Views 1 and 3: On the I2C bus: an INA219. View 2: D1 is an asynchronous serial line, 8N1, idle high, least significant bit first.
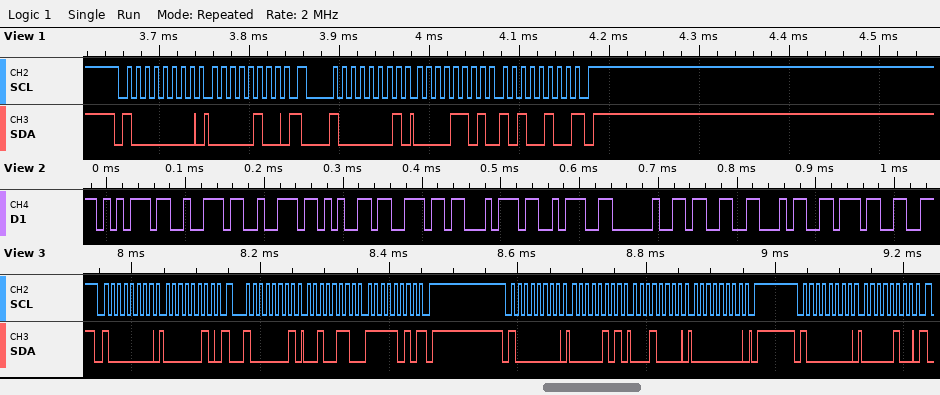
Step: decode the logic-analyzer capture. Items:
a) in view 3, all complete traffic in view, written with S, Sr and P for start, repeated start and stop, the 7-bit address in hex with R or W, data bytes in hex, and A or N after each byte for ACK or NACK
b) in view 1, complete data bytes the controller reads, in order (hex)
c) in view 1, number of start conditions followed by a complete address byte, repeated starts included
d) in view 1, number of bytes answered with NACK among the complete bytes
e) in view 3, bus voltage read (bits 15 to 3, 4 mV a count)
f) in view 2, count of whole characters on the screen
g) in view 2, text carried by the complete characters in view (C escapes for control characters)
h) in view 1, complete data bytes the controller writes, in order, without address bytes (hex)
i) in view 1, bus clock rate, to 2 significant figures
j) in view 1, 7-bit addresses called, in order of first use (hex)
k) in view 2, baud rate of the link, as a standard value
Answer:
S 40W A 02 A Sr 40R A 26 A FA N P S 40W A 05 A 10 A 00 A P S 40W A 04 A
0D A4
2
1
4.988 V
11
"urrent: 347"
04
100 kHz
0x40
115200 baud
